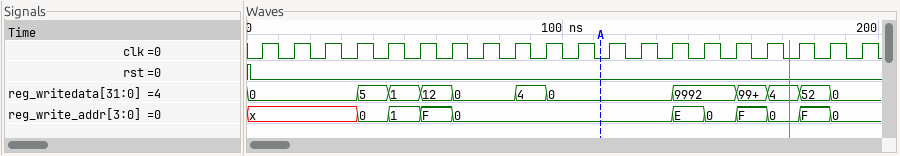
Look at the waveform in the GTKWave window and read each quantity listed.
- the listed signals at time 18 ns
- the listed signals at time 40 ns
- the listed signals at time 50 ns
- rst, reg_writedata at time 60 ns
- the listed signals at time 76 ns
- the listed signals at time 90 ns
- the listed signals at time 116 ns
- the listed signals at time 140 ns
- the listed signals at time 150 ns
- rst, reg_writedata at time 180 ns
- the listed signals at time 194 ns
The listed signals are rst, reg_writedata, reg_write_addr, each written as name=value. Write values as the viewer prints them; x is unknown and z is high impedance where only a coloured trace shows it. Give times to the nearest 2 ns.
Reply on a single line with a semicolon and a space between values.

rst=0, reg_writedata=0, reg_write_addr=x; rst=0, reg_writedata=5, reg_write_addr=0; rst=0, reg_writedata=1, reg_write_addr=1; rst=0, reg_writedata=12; rst=0, reg_writedata=0, reg_write_addr=0; rst=0, reg_writedata=4, reg_write_addr=0; rst=0, reg_writedata=0, reg_write_addr=0; rst=0, reg_writedata=9992, reg_write_addr=E; rst=0, reg_writedata=9992, reg_write_addr=0; rst=0, reg_writedata=52; rst=0, reg_writedata=0, reg_write_addr=0
